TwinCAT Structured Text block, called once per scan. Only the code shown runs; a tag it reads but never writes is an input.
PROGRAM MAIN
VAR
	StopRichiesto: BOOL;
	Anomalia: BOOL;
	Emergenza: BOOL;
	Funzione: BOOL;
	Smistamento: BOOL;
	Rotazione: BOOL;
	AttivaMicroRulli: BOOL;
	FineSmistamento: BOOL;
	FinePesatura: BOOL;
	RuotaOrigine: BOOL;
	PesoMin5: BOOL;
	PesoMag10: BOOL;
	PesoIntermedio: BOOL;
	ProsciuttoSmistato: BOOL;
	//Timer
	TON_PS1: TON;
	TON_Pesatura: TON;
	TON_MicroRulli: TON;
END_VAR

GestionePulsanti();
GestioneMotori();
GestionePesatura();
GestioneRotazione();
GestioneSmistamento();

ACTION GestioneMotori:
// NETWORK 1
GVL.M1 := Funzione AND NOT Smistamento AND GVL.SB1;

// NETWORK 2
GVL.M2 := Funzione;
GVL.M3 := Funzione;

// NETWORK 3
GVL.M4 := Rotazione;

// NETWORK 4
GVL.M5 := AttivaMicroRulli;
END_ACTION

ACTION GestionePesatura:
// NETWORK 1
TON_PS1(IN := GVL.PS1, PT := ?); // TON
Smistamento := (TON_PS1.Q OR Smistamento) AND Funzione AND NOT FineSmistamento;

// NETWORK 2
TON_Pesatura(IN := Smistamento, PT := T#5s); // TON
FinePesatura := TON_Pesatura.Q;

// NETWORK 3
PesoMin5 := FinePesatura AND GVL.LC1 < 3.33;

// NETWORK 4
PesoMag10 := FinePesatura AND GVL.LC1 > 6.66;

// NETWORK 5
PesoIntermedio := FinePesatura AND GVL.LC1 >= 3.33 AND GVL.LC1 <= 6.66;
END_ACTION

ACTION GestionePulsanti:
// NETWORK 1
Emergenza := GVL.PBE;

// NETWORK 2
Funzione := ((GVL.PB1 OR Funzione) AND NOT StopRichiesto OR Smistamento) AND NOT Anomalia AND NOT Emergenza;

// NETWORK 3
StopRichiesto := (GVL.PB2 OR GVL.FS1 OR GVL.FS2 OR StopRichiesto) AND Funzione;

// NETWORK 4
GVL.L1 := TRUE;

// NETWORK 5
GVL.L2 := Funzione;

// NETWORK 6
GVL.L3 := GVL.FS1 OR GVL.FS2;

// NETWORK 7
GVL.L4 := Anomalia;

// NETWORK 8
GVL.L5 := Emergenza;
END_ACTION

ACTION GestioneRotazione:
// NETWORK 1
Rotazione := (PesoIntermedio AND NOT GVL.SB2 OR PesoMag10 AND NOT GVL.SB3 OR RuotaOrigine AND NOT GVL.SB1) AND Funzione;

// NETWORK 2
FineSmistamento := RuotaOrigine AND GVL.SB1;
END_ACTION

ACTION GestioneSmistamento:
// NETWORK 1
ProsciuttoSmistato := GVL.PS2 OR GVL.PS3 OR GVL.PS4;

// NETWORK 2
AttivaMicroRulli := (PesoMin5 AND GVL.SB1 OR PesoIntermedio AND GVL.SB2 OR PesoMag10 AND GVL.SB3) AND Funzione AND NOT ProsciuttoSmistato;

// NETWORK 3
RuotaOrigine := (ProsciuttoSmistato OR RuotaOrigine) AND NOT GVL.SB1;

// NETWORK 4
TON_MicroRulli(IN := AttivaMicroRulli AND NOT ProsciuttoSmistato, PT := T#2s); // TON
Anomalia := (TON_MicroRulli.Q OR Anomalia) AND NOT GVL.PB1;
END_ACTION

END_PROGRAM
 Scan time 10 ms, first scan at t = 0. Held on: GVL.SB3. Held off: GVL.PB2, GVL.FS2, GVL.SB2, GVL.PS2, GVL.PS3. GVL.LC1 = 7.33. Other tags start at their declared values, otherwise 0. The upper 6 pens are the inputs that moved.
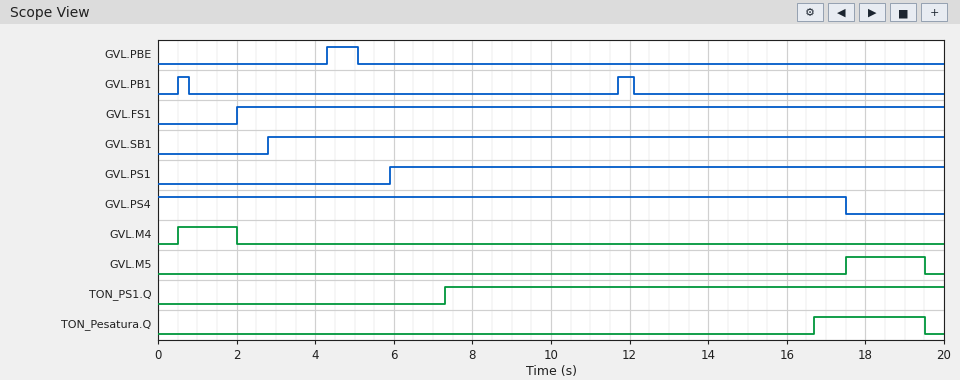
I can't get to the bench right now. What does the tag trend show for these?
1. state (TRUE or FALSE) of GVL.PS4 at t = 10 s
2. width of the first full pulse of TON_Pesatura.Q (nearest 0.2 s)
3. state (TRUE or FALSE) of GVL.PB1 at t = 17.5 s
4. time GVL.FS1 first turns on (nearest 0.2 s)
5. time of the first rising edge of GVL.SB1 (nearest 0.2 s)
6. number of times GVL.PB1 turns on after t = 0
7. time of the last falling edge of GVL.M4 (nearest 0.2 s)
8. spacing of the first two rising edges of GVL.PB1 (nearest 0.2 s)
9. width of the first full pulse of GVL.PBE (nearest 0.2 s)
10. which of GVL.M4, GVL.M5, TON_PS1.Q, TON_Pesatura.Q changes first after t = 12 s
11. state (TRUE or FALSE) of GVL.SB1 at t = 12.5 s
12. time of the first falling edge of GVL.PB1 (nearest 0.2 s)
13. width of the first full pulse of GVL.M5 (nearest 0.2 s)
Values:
TRUE
2.8 s
FALSE
2.0 s
2.8 s
2
2.0 s
11.2 s
0.8 s
TON_Pesatura.Q
TRUE
0.8 s
2.0 s
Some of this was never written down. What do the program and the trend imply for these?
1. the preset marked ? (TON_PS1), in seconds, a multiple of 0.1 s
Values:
1.4 s
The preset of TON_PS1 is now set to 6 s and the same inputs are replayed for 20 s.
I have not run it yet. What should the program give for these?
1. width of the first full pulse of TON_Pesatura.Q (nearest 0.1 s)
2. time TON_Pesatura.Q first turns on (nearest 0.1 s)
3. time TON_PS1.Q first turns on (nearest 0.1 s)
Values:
2.6 s
16.9 s
11.9 s
